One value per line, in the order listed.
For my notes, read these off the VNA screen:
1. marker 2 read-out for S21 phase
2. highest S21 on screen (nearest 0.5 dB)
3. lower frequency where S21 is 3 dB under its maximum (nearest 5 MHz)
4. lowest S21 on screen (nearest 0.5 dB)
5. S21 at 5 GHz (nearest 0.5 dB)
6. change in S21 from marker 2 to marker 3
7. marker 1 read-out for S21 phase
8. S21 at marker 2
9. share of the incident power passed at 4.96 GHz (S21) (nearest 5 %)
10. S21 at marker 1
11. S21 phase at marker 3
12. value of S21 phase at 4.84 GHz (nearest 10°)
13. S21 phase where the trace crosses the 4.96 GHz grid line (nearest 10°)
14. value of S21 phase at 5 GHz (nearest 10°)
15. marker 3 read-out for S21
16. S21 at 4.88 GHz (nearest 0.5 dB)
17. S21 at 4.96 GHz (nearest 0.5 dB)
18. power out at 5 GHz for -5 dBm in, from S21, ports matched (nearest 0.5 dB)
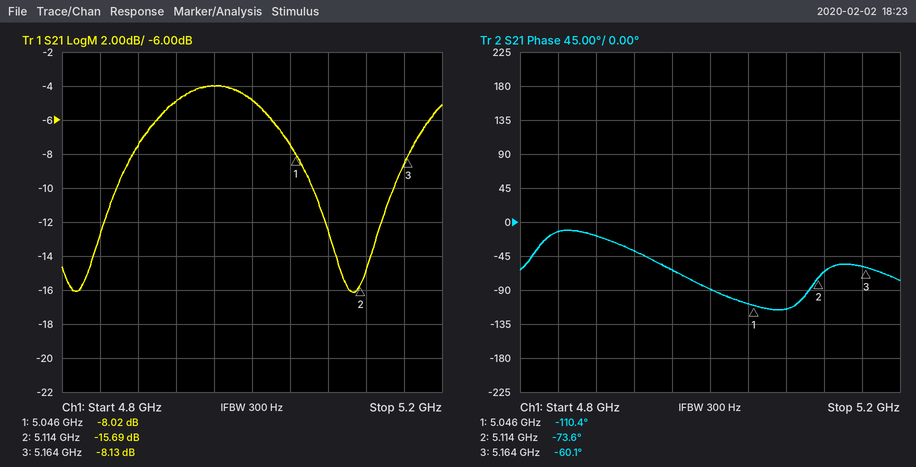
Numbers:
-73.6°
-4.0 dB
4.885 GHz
-16.0 dB
-5.0 dB
7.56 dB
-110.4°
-15.69 dB
40 %
-8.02 dB
-60.1°
-10°
-60°
-90°
-8.13 dB
-7.5 dB
-4.0 dB
-10.0 dBm
